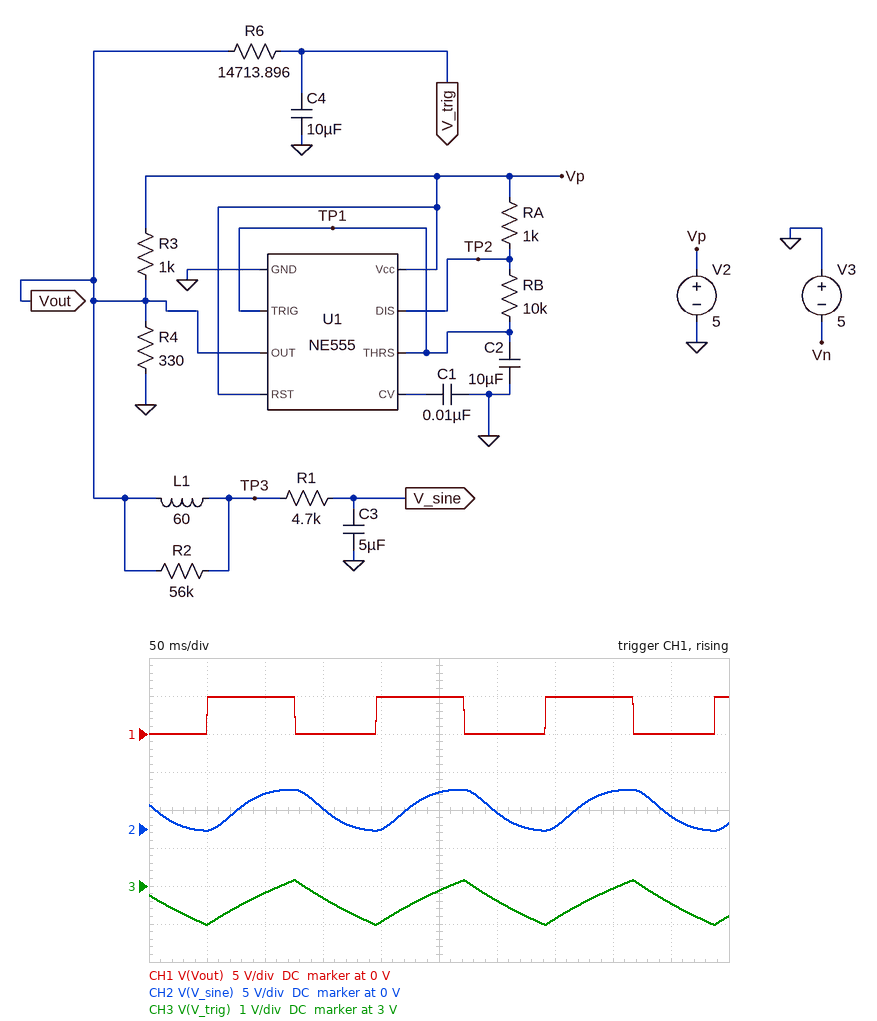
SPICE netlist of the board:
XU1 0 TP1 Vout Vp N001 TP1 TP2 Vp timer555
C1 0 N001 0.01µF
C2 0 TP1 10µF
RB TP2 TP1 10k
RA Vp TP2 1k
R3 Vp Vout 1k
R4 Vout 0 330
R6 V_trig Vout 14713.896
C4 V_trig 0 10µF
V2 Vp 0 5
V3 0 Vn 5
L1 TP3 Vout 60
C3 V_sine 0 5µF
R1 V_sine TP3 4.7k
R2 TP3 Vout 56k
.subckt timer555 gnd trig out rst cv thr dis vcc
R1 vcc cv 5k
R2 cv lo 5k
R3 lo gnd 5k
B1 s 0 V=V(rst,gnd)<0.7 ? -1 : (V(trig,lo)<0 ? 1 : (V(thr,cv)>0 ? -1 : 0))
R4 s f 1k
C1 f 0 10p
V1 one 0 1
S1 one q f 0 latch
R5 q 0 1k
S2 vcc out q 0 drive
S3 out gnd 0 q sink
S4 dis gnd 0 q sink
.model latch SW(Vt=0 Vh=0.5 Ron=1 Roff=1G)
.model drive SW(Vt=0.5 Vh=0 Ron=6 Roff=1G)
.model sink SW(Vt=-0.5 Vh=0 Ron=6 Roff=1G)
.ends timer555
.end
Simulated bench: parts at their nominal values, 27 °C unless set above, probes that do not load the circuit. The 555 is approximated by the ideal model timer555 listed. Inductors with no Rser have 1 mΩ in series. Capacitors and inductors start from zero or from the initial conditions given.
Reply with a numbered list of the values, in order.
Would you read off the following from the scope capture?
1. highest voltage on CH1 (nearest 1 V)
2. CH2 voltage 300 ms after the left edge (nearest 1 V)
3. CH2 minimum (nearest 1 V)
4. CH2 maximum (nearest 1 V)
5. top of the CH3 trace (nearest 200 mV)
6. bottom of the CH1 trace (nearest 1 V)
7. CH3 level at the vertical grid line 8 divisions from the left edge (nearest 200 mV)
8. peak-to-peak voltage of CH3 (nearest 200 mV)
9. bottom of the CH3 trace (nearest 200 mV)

1. 5 V
2. 2 V
3. 0 V
4. 5 V
5. 3.2 V
6. 0 V
7. 3.0 V
8. 1.2 V
9. 2.0 V
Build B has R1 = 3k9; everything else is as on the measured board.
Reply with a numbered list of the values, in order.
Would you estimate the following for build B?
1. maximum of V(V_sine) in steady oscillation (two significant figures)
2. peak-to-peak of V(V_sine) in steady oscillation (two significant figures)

1. 5.5 V
2. 6.1 V
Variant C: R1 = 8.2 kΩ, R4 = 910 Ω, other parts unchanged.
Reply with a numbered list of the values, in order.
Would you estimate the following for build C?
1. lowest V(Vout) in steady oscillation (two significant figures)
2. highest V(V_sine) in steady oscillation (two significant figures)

1. 31 mV
2. 4.4 V
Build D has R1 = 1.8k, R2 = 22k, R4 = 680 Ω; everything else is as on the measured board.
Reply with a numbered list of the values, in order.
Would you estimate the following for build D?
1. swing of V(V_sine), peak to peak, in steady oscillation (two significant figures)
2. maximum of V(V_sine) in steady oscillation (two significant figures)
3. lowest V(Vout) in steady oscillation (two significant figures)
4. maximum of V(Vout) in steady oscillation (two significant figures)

1. 9.4 V
2. 7.2 V
3. 28 mV
4. 5.0 V
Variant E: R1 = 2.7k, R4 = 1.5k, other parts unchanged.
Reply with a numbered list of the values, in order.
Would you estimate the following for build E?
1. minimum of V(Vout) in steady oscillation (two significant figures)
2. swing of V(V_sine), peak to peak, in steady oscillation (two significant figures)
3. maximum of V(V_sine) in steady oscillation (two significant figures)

1. 29 mV
2. 7.9 V
3. 6.5 V
